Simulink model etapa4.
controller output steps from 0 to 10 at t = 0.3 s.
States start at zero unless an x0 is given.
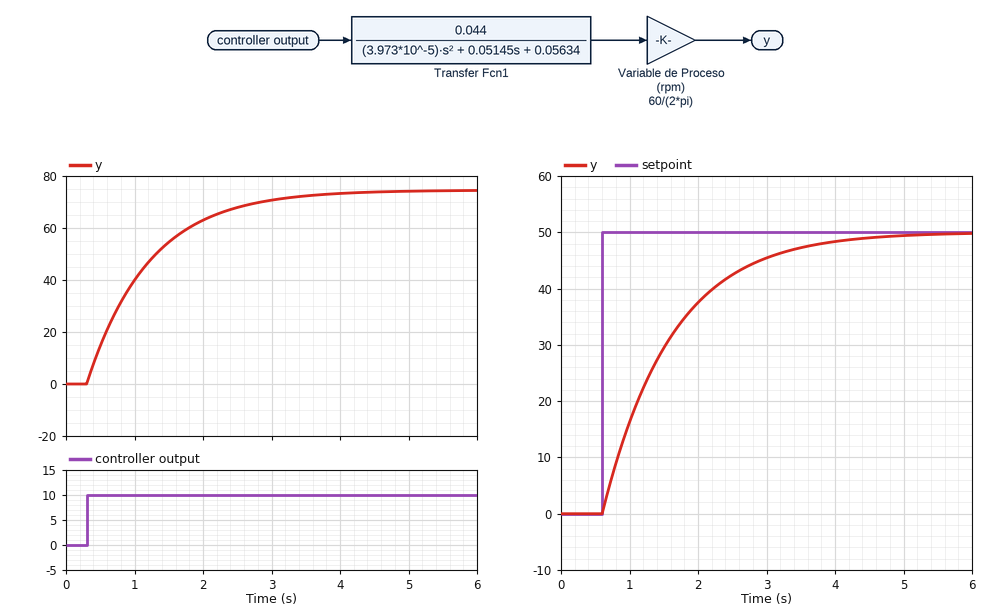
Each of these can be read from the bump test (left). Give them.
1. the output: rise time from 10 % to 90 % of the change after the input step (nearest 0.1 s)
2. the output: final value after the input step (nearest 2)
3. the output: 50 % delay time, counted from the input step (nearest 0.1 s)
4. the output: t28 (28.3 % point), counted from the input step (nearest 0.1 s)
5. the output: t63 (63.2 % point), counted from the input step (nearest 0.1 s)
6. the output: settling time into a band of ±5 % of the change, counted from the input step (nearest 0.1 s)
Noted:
2.0 s
74
0.6 s
0.3 s
0.9 s
2.7 s
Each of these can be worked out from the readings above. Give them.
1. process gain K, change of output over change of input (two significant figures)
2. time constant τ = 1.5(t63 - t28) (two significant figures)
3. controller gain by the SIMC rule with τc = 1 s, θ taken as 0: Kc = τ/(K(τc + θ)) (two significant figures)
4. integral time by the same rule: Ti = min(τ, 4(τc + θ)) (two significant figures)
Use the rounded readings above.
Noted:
7.4
0.90 s
0.12
0.90 s
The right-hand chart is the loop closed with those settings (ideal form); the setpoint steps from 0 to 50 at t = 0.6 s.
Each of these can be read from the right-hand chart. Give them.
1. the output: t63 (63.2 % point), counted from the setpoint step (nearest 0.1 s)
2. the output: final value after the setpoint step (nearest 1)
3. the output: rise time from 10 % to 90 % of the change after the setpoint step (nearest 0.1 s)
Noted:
1.0 s
50
2.2 s
